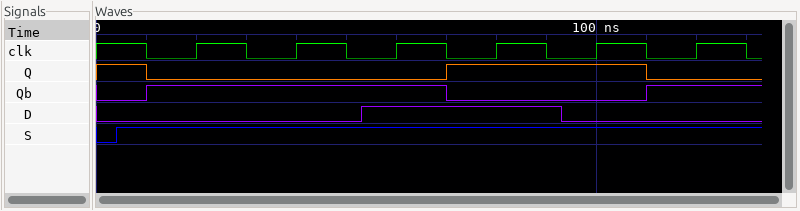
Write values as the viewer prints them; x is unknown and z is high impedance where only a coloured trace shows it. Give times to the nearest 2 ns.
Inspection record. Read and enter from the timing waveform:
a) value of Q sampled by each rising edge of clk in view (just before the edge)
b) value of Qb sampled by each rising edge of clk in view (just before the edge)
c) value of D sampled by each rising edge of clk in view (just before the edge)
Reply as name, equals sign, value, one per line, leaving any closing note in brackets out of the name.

value of Q sampled by each rising edge of clk in view = 0 0 0 1 1 0
value of Qb sampled by each rising edge of clk in view = 1 1 1 0 0 1
value of D sampled by each rising edge of clk in view = 0 0 1 1 0 0
